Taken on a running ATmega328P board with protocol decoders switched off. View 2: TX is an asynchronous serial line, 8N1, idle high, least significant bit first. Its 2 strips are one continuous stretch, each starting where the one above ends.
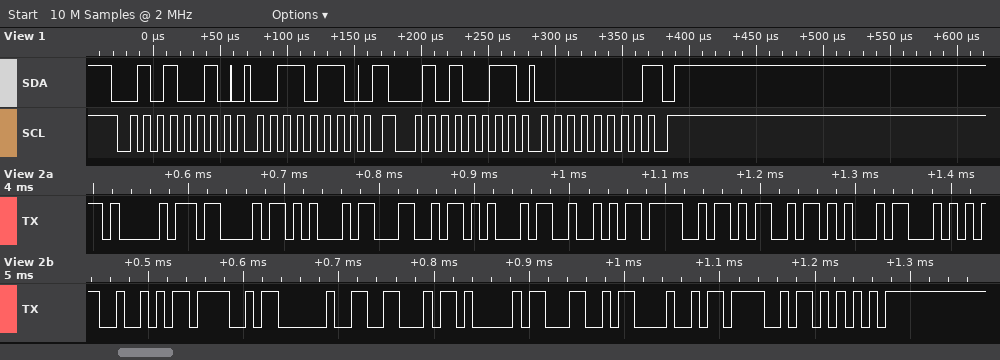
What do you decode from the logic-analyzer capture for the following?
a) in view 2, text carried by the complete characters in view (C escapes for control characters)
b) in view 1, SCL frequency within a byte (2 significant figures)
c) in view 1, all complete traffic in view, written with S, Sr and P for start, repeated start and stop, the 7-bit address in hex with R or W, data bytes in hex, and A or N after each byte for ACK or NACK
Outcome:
"ACELEROMETRO FALHOU"
100 kHz
S 29W A 36 A Sr 29R A 00 N P
